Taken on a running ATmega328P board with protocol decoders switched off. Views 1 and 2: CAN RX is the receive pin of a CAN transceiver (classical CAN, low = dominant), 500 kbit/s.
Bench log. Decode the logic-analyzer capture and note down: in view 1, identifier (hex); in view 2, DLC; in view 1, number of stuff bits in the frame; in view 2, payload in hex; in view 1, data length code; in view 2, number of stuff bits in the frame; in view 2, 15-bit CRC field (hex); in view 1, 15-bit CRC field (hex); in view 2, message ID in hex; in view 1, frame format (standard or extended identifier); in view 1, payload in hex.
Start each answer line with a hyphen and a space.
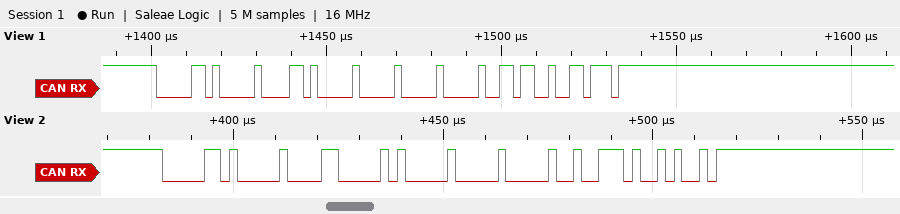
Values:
- 0x050
- 3
- 6
- 02 00 00
- 3
- 6
- 0x4E94
- 0x6C9B
- 0x050
- standard
- 40 00 00
